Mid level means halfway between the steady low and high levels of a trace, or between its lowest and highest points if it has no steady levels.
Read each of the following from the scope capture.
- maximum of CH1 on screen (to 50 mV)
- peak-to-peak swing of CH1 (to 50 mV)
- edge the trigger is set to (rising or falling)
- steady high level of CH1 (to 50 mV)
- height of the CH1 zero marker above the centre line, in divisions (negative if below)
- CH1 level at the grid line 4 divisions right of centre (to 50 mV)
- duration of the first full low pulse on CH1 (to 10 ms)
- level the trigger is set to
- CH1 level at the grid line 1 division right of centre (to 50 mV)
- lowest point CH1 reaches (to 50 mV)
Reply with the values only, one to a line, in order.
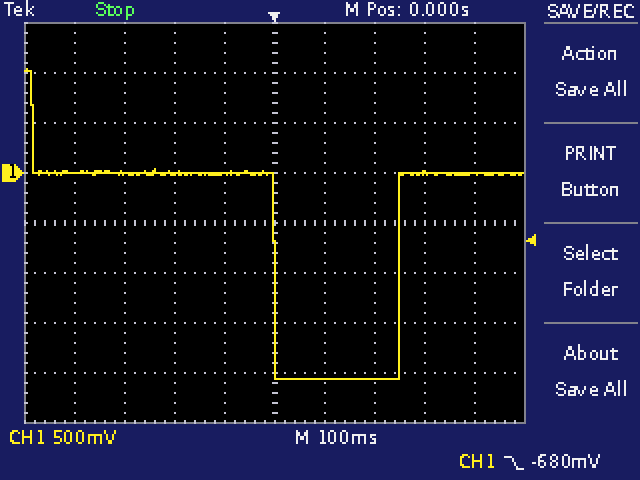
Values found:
1.05 V
3.10 V
falling
0 mV
+1.0 div
0 mV
250 ms
-680 mV
-2.05 V
-2.05 V
